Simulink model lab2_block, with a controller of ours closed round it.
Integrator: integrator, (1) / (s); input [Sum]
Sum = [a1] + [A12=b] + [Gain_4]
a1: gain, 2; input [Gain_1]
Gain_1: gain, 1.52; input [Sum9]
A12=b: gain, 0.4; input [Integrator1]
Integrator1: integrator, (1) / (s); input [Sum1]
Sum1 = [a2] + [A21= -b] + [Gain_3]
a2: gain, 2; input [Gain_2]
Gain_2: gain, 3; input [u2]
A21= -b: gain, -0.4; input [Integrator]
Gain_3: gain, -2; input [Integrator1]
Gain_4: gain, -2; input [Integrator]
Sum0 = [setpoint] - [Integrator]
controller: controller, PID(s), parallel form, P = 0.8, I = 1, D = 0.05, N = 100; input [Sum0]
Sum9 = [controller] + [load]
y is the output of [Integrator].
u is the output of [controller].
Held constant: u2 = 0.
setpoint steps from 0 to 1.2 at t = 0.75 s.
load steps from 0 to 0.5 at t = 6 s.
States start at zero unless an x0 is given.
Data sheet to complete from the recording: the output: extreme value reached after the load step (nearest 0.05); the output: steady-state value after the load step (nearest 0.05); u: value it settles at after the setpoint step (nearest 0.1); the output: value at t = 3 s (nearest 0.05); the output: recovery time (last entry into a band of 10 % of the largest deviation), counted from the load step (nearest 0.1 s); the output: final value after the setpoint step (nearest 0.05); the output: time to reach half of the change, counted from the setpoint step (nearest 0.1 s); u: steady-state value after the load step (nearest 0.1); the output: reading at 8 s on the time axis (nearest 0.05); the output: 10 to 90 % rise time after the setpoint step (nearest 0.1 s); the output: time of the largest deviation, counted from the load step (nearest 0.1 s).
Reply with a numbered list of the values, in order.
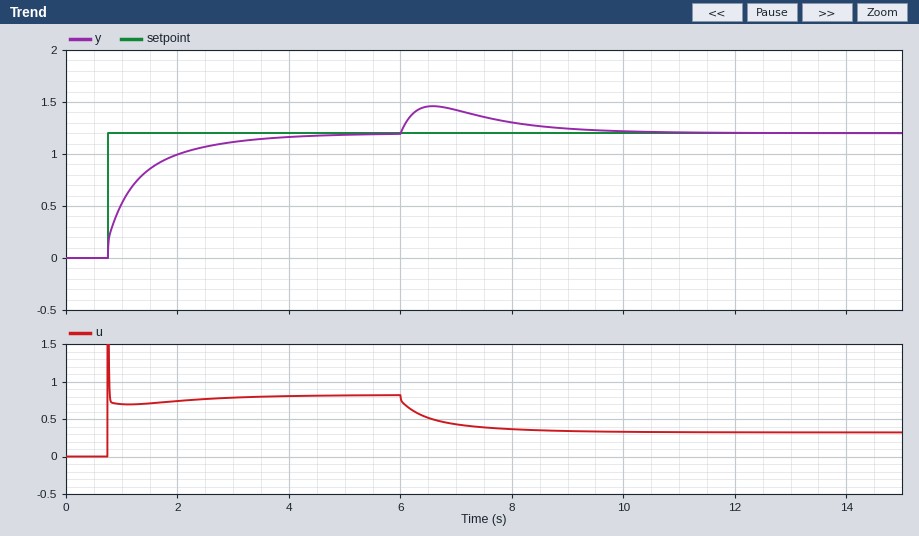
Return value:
1. 1.45
2. 1.20
3. 0.8
4. 1.10
5. 3.6 s
6. 1.20
7. 0.3 s
8. 0.3
9. 1.30
10. 1.8 s
11. 0.6 s
